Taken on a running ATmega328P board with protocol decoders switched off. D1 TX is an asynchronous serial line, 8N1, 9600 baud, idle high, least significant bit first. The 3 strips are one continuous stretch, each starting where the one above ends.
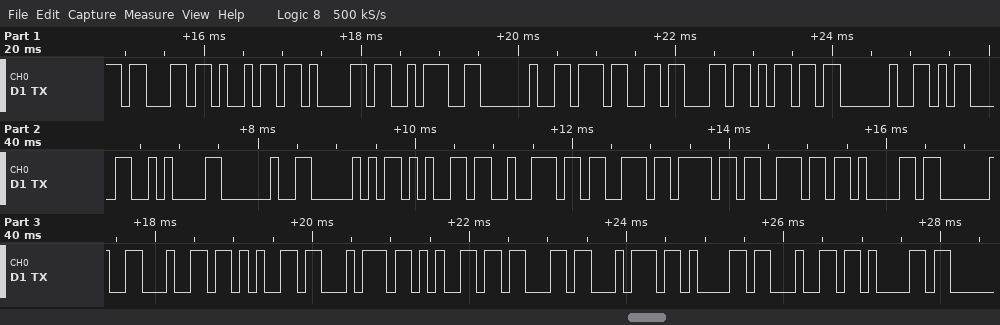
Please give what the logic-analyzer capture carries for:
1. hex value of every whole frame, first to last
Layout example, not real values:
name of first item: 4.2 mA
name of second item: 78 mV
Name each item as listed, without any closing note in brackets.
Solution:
hex value of every whole frame, first to last: 63 69 61 3A 20 37 63 6D 20 0D 0A 20 50 65 72 73 6F 6E 61 20 64 65 74 65 63 74 61 64 61
